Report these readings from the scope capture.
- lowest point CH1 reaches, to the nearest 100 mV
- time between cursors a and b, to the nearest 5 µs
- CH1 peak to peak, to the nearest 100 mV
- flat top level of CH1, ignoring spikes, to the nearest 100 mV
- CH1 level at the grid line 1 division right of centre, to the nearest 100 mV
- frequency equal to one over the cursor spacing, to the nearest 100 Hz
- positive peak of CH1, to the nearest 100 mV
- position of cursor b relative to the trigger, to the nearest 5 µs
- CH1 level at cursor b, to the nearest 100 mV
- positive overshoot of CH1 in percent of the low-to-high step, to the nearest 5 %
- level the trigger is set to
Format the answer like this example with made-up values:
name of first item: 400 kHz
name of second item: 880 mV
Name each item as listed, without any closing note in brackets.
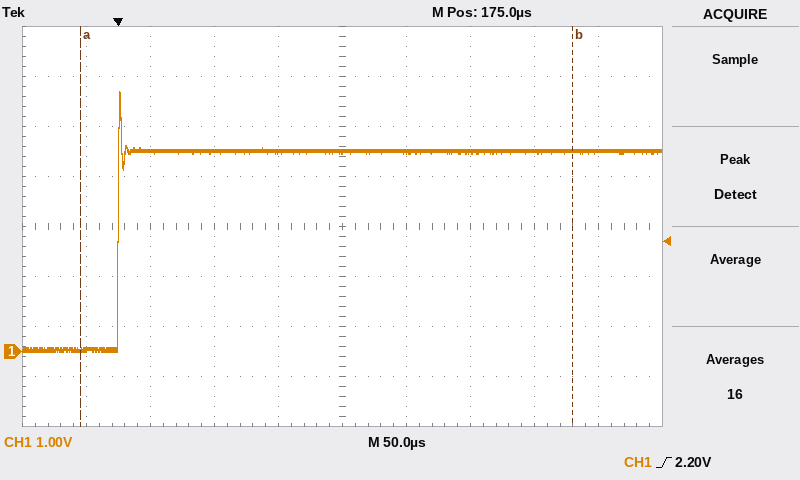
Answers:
lowest point CH1 reaches, to the nearest 100 mV: 0.0 V
time between cursors a and b, to the nearest 5 µs: 385 µs
CH1 peak to peak, to the nearest 100 mV: 5.2 V
flat top level of CH1, ignoring spikes, to the nearest 100 mV: 4.0 V
CH1 level at the grid line 1 division right of centre, to the nearest 100 mV: 4.0 V
frequency equal to one over the cursor spacing, to the nearest 100 Hz: 2.6 kHz
positive peak of CH1, to the nearest 100 mV: 5.2 V
position of cursor b relative to the trigger, to the nearest 5 µs: +355 µs
CH1 level at cursor b, to the nearest 100 mV: 4.0 V
positive overshoot of CH1 in percent of the low-to-high step, to the nearest 5 %: 30 %
level the trigger is set to: 2.20 V
